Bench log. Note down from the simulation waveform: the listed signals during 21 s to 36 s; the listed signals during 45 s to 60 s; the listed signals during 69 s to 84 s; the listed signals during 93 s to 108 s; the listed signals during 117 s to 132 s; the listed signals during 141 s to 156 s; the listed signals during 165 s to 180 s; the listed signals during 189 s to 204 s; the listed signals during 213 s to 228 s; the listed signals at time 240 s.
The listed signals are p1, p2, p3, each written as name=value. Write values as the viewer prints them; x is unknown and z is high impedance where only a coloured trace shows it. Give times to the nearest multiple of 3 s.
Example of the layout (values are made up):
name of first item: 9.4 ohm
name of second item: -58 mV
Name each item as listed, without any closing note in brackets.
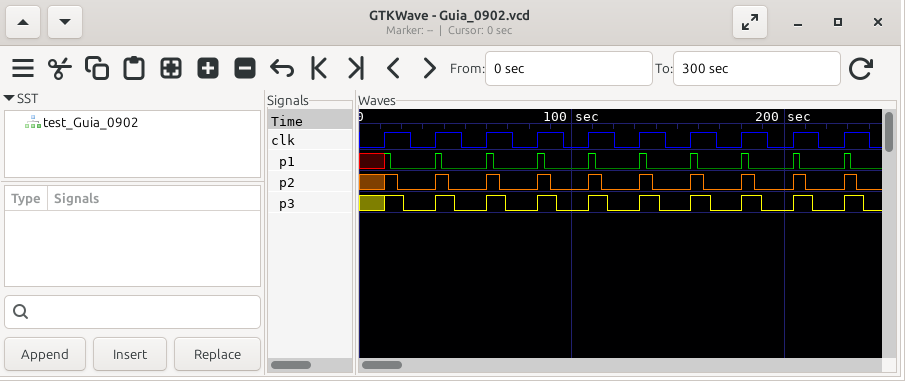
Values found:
the listed signals during 21 s to 36 s: p1=0, p2=0, p3=0
the listed signals during 45 s to 60 s: p1=0, p2=0, p3=0
the listed signals during 69 s to 84 s: p1=0, p2=0, p3=0
the listed signals during 93 s to 108 s: p1=0, p2=0, p3=0
the listed signals during 117 s to 132 s: p1=0, p2=0, p3=0
the listed signals during 141 s to 156 s: p1=0, p2=0, p3=0
the listed signals during 165 s to 180 s: p1=0, p2=0, p3=0
the listed signals during 189 s to 204 s: p1=0, p2=0, p3=0
the listed signals during 213 s to 228 s: p1=0, p2=0, p3=0
the listed signals at time 240 s: p1=0, p2=0, p3=0
